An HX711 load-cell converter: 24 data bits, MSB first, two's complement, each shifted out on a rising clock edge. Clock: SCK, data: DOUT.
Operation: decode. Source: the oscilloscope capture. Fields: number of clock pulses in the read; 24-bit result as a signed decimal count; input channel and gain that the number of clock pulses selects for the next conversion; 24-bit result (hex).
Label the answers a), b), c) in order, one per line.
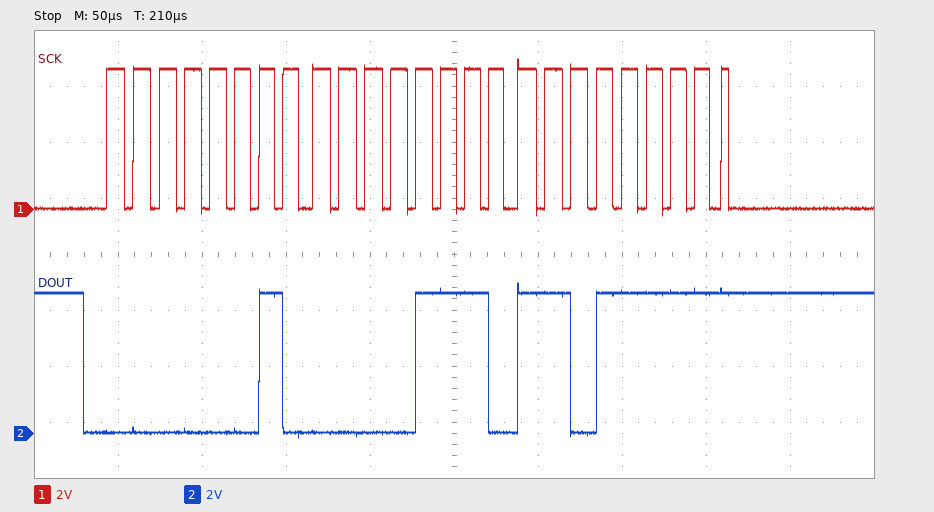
a) 25
b) 134879
c) channel A, gain 128
d) 0x020EDF
